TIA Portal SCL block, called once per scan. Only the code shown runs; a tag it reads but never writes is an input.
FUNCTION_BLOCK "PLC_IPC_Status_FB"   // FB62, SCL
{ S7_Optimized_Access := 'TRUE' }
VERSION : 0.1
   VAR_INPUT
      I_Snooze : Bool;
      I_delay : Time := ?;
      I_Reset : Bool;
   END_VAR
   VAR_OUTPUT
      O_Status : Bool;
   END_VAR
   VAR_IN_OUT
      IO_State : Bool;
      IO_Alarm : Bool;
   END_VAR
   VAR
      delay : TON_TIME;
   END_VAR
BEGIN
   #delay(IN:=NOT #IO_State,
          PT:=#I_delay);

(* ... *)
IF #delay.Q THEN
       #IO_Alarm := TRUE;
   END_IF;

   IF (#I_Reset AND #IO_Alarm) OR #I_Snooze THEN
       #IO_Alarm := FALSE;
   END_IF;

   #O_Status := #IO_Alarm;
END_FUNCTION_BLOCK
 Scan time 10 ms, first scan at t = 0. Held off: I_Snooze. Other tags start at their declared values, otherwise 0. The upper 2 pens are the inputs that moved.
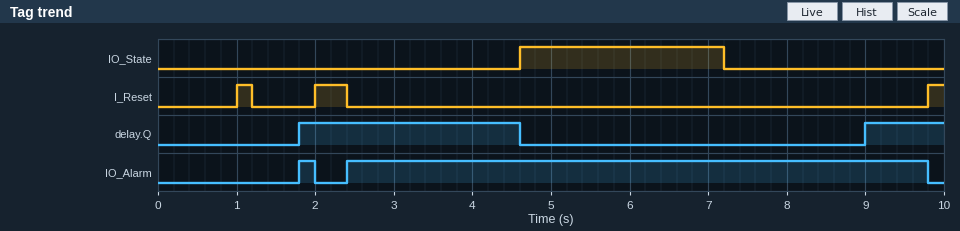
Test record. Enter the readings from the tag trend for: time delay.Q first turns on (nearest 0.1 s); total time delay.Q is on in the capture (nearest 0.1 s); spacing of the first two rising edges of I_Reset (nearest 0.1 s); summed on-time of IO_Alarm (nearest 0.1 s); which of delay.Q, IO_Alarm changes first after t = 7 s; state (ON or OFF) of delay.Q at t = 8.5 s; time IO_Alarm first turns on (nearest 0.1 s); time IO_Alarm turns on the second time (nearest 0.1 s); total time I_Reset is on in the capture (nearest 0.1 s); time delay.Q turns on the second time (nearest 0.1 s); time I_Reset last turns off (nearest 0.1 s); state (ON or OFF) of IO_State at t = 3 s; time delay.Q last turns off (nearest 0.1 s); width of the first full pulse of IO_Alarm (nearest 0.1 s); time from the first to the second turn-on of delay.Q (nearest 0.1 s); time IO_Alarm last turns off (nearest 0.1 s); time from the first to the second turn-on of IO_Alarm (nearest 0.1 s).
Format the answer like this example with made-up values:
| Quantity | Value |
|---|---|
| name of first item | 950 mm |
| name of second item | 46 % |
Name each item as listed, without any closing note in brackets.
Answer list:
| Quantity | Value |
|---|---|
| time delay.Q first turns on | 1.8 s |
| total time delay.Q is on in the capture | 3.8 s |
| spacing of the first two rising edges of I_Reset | 1.0 s |
| summed on-time of IO_Alarm | 7.6 s |
| which of delay.Q, IO_Alarm changes first after t = 7 s | delay.Q |
| state (ON or OFF) of delay.Q at t = 8.5 s | OFF |
| time IO_Alarm first turns on | 1.8 s |
| time IO_Alarm turns on the second time | 2.4 s |
| total time I_Reset is on in the capture | 0.8 s |
| time delay.Q turns on the second time | 9.0 s |
| time I_Reset last turns off | 2.4 s |
| state (ON or OFF) of IO_State at t = 3 s | OFF |
| time delay.Q last turns off | 4.6 s |
| width of the first full pulse of IO_Alarm | 0.2 s |
| time from the first to the second turn-on of delay.Q | 7.2 s |
| time IO_Alarm last turns off | 9.8 s |
| time from the first to the second turn-on of IO_Alarm | 0.6 s |
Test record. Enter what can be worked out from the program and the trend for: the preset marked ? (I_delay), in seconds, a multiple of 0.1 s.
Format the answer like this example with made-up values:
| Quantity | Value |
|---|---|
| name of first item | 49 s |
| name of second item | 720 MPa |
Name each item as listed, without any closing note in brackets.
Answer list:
| Quantity | Value |
|---|---|
| the preset marked ? (I_delay), in seconds, a multiple of 0.1 s | 1.8 s |
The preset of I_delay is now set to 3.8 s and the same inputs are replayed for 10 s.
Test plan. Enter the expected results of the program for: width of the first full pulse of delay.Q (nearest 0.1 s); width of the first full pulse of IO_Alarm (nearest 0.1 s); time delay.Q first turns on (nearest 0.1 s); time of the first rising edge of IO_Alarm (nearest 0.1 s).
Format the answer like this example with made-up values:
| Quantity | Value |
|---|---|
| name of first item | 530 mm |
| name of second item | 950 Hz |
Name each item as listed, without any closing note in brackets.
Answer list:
| Quantity | Value |
|---|---|
| width of the first full pulse of delay.Q | 0.8 s |
| width of the first full pulse of IO_Alarm | 6.0 s |
| time delay.Q first turns on | 3.8 s |
| time of the first rising edge of IO_Alarm | 3.8 s |
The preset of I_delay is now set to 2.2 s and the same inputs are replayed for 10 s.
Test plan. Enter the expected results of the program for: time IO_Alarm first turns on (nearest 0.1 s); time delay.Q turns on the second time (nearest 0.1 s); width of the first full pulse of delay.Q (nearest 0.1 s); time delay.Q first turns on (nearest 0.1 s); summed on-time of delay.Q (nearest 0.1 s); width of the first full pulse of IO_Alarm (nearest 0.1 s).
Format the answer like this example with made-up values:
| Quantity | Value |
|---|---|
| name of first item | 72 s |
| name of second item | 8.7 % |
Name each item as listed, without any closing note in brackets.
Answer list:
| Quantity | Value |
|---|---|
| time IO_Alarm first turns on | 2.4 s |
| time delay.Q turns on the second time | 9.4 s |
| width of the first full pulse of delay.Q | 2.4 s |
| time delay.Q first turns on | 2.2 s |
| summed on-time of delay.Q | 3.0 s |
| width of the first full pulse of IO_Alarm | 7.4 s |
